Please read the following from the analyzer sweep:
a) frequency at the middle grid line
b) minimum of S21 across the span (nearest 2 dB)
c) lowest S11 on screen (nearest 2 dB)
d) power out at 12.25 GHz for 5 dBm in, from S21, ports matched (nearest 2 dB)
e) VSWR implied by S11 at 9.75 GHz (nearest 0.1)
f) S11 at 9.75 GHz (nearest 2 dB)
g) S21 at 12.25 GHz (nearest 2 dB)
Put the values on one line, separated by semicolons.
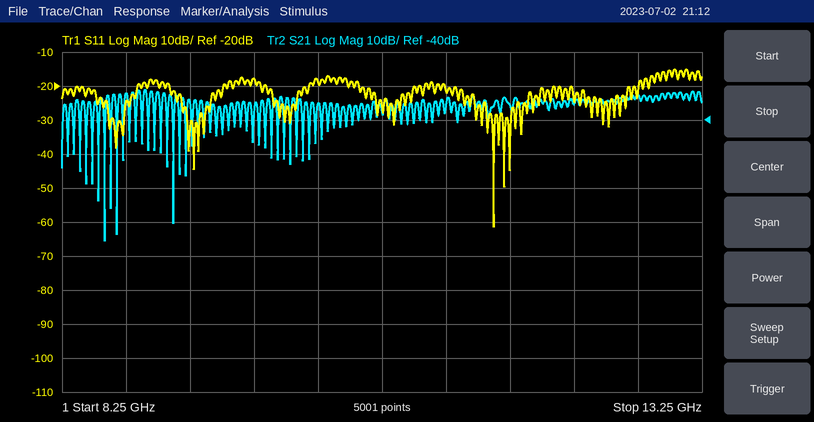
10.75 GHz; -76 dB; -62 dB; -30 dBm; 1.3; -18 dB; -36 dB
